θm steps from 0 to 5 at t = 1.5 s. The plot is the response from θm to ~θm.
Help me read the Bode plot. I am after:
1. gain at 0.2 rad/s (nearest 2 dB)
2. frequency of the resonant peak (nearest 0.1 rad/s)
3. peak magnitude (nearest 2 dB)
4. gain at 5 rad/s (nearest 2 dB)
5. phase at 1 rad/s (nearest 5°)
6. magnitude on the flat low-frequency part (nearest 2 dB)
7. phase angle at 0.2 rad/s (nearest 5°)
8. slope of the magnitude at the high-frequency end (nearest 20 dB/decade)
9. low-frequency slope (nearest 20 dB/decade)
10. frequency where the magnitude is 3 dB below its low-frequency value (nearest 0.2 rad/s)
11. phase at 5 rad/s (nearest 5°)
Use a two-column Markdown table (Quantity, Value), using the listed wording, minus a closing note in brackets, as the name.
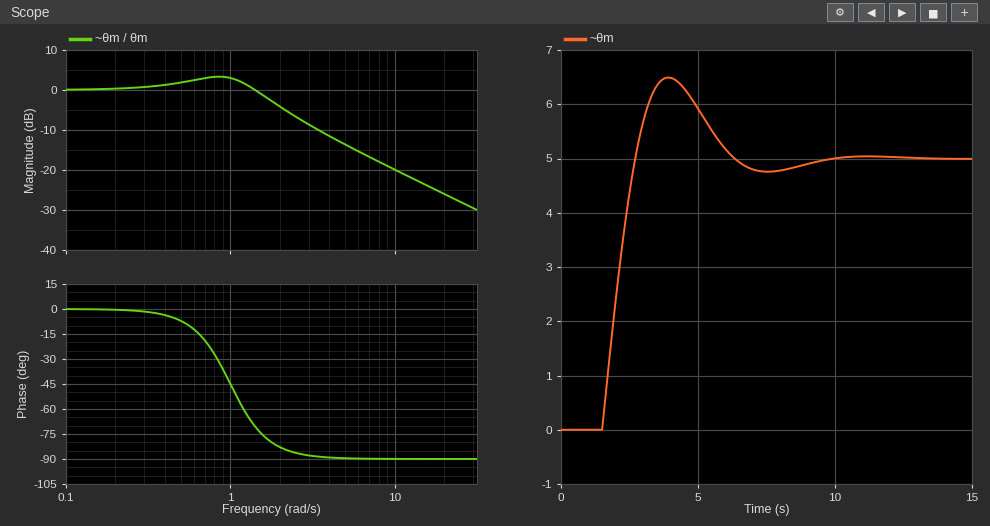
| Quantity | Value |
|---|---|
| gain at 0.2 rad/s | 0 dB |
| frequency of the resonant peak | 0.8 rad/s |
| peak magnitude | 4 dB |
| gain at 5 rad/s | -14 dB |
| phase at 1 rad/s | -45° |
| magnitude on the flat low-frequency part | 0 dB |
| phase angle at 0.2 rad/s | 0° |
| slope of the magnitude at the high-frequency end | -20 dB/decade |
| low-frequency slope | 0 dB/decade |
| frequency where the magnitude is 3 dB below its low-frequency value | 1.8 rad/s |
| phase at 5 rad/s | -90° |
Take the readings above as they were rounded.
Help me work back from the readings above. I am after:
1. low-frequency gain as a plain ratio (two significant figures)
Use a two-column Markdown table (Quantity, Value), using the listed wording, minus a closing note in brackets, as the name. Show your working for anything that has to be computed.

| Quantity | Value |
|---|---|
| low-frequency gain as a plain ratio | 10^(0 / 20) = 1.0 |
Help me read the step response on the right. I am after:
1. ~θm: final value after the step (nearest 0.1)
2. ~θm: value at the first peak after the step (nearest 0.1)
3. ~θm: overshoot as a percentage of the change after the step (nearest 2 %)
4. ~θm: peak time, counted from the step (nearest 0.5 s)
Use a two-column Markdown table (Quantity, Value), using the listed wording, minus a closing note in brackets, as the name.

| Quantity | Value |
|---|---|
| ~θm: final value after the step | 5.0 |
| ~θm: value at the first peak after the step | 6.5 |
| ~θm: overshoot as a percentage of the change after the step | 30 % |
| ~θm: peak time, counted from the step | 2.5 s |
